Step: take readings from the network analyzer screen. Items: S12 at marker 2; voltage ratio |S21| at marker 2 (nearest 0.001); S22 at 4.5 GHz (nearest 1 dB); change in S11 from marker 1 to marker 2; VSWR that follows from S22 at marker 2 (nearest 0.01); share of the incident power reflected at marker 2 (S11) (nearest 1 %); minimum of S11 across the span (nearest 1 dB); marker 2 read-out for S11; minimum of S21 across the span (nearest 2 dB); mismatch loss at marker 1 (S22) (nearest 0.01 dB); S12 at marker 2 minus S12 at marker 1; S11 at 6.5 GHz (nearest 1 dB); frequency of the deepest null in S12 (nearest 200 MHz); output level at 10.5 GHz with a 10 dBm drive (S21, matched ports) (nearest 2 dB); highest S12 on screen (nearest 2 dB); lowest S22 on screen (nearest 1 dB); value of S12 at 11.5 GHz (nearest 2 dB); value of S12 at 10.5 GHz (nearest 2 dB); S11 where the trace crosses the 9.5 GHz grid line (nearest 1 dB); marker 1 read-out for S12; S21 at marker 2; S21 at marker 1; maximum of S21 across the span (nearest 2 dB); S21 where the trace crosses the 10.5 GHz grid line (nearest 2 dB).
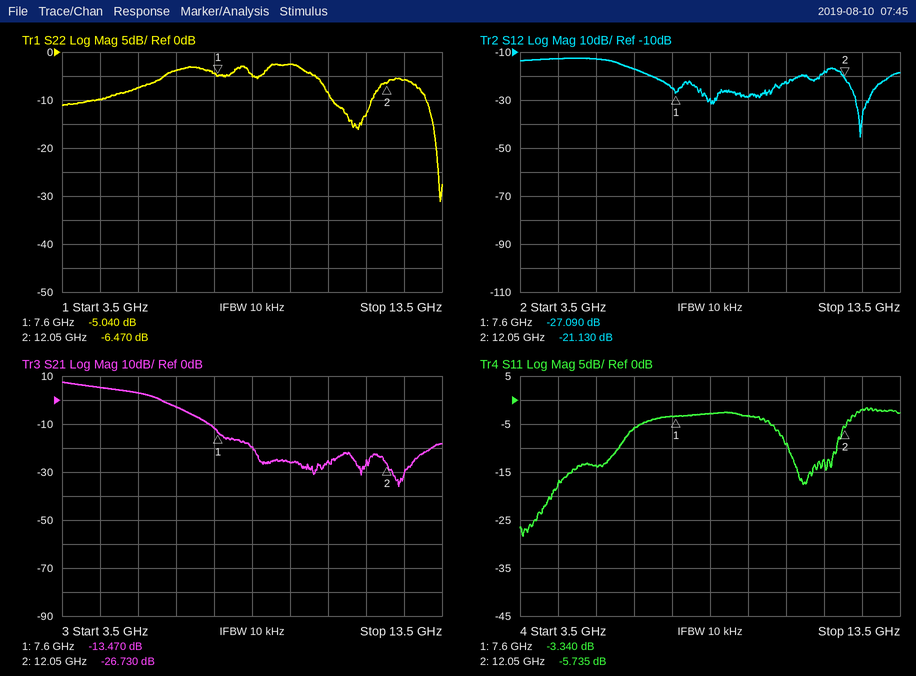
-21.130 dB
0.046
-10 dB
-2.395 dB
2.81
27 %
-28 dB
-5.735 dB
-36 dB
1.63 dB
5.960 dB
-6 dB
12.4 GHz
-16 dBm
-12 dB
-31 dB
-18 dB
-22 dB
-3 dB
-27.090 dB
-26.730 dB
-13.470 dB
8 dB
-26 dB
